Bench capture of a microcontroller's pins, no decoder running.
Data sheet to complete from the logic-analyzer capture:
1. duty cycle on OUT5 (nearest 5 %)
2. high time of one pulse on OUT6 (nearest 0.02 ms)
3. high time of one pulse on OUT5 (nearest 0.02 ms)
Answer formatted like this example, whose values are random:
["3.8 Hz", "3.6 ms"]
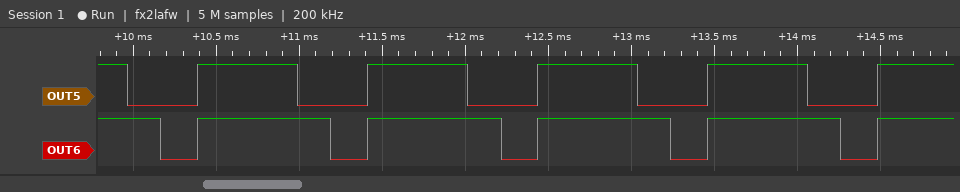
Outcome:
["60 %", "0.80 ms", "0.60 ms"]
